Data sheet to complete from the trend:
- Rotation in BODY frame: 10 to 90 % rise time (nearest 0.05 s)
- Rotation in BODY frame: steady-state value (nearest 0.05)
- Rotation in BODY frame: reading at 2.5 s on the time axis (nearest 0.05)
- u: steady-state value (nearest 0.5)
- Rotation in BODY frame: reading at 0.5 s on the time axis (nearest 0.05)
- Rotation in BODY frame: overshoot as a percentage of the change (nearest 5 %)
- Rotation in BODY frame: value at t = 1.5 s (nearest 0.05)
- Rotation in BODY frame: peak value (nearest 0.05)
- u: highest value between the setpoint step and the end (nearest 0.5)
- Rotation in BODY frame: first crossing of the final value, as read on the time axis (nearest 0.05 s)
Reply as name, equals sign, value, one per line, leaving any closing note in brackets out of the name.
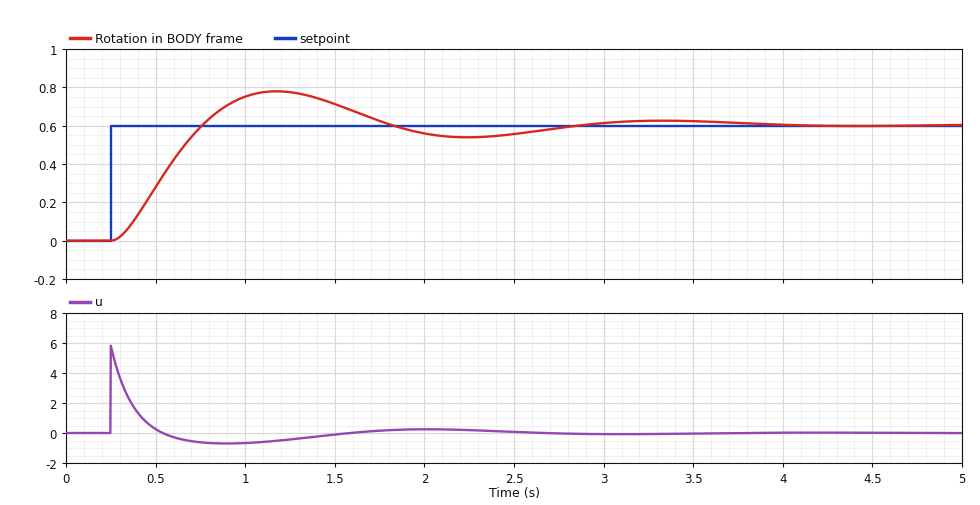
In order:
Rotation in BODY frame: 10 to 90 % rise time = 0.35 s
Rotation in BODY frame: steady-state value = 0.60
Rotation in BODY frame: reading at 2.5 s on the time axis = 0.55
u: steady-state value = 0.0
Rotation in BODY frame: reading at 0.5 s on the time axis = 0.30
Rotation in BODY frame: overshoot as a percentage of the change = 30 %
Rotation in BODY frame: value at t = 1.5 s = 0.70
Rotation in BODY frame: peak value = 0.80
u: highest value between the setpoint step and the end = 6.0
Rotation in BODY frame: first crossing of the final value, as read on the time axis = 0.75 s
